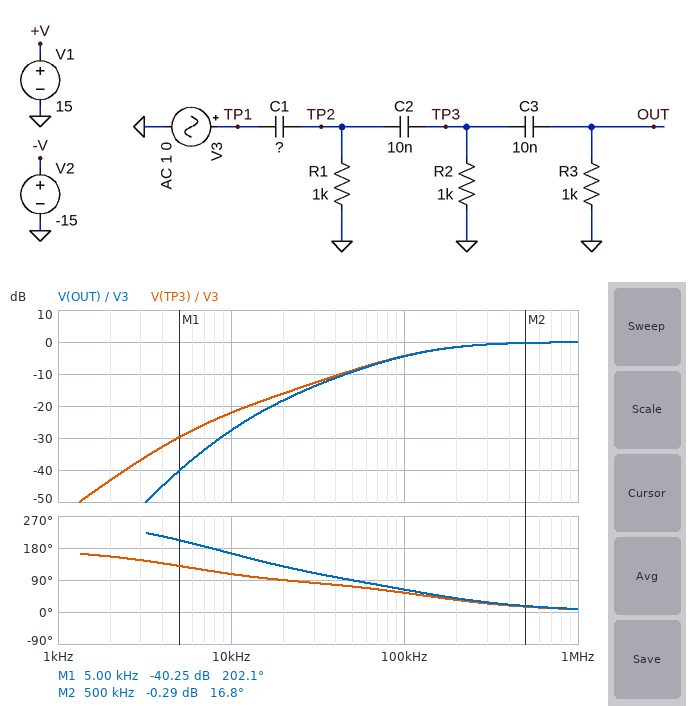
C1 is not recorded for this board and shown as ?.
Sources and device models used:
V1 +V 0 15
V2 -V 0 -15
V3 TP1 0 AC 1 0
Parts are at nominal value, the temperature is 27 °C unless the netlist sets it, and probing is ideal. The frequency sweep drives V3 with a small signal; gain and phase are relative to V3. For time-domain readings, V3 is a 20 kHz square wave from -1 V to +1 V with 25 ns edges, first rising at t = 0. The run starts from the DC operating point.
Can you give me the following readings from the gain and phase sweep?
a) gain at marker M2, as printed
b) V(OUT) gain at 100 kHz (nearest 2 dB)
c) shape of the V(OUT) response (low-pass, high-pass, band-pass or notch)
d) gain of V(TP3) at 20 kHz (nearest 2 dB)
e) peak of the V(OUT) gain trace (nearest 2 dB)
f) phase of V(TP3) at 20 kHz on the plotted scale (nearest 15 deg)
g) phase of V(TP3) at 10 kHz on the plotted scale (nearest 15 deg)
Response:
-0.29 dB
-4 dB
high-pass
-16 dB
0 dB
90 deg
105 deg
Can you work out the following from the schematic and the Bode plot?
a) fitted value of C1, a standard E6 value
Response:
4.7 nF
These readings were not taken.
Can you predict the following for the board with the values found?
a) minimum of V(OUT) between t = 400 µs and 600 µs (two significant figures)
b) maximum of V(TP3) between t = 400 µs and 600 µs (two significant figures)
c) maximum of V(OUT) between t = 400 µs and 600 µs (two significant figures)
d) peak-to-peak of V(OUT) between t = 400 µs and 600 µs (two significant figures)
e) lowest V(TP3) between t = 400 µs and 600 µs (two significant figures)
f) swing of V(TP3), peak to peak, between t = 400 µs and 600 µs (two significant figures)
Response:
-2.0 V
2.0 V
2.0 V
4.0 V
-2.0 V
4.0 V
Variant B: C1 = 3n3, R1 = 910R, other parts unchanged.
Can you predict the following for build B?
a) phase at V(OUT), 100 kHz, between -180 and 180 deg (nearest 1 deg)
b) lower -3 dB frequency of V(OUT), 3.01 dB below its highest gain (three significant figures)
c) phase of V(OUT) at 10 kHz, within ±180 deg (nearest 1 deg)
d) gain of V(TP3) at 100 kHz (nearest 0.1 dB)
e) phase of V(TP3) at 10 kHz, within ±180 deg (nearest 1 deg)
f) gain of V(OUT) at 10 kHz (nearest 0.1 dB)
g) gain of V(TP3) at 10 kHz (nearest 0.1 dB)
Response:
72 deg
179 kHz
170 deg
-6.2 dB
112 deg
-30.9 dB
-25.4 dB
